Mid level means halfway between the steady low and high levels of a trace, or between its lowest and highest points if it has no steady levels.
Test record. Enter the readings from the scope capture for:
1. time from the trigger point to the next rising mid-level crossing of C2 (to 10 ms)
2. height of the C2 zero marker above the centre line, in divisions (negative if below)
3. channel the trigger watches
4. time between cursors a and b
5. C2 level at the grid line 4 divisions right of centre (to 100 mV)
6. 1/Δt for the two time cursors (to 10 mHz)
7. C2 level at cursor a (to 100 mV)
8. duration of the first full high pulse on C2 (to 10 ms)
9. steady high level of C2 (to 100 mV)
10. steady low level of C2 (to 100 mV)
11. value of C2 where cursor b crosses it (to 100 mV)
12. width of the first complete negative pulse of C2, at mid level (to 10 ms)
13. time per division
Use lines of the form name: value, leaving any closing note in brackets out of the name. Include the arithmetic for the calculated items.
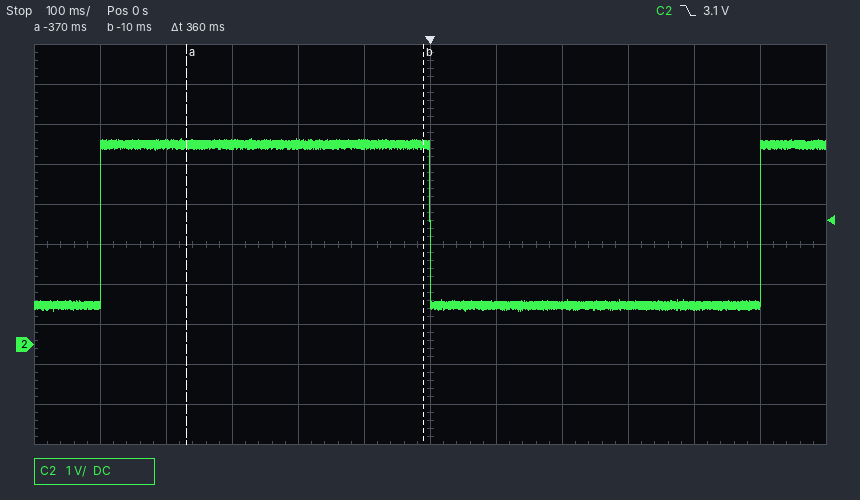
time from the trigger point to the next rising mid-level crossing of C2: 500 ms
height of the C2 zero marker above the centre line, in divisions: -2.5 div
channel the trigger watches: C2
time between cursors a and b: 360 ms
C2 level at the grid line 4 divisions right of centre: 1.0 V
1/Δt for the two time cursors: 1 / 360 ms ≈ 2.78 Hz
C2 level at cursor a: 5.0 V
duration of the first full high pulse on C2: 500 ms
steady high level of C2: 5.0 V
steady low level of C2: 1.0 V
value of C2 where cursor b crosses it: 5.0 V
width of the first complete negative pulse of C2, at mid level: 500 ms
time per division: 100 ms
